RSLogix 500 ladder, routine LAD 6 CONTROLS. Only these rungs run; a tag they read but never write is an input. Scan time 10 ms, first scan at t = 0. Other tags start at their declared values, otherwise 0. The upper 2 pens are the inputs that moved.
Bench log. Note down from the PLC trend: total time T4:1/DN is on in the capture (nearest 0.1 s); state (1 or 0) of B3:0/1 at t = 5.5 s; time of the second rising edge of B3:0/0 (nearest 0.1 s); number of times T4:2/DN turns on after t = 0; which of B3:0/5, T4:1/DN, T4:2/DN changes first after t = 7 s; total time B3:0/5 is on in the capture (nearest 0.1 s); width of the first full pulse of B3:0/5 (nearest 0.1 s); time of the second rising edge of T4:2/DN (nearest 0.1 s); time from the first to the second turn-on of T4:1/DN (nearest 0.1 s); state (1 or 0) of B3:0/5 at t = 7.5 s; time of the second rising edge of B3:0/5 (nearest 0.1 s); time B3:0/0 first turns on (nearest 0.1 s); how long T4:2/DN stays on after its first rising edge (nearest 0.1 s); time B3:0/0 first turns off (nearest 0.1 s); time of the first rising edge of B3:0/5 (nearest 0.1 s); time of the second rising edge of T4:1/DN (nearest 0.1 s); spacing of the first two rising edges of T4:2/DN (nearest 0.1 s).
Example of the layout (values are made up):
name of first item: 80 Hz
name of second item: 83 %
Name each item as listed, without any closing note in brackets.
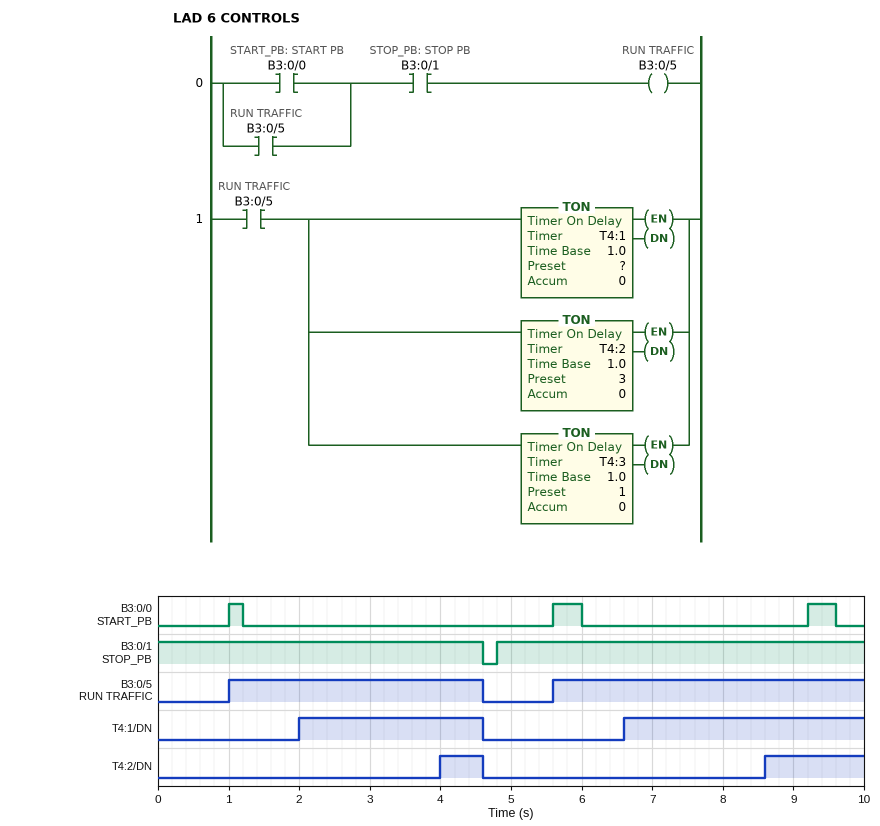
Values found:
total time T4:1/DN is on in the capture: 6.0 s
state (1 or 0) of B3:0/1 at t = 5.5 s: 1
time of the second rising edge of B3:0/0: 5.6 s
number of times T4:2/DN turns on after t = 0: 2
which of B3:0/5, T4:1/DN, T4:2/DN changes first after t = 7 s: T4:2/DN
total time B3:0/5 is on in the capture: 8.0 s
width of the first full pulse of B3:0/5: 3.6 s
time of the second rising edge of T4:2/DN: 8.6 s
time from the first to the second turn-on of T4:1/DN: 4.6 s
state (1 or 0) of B3:0/5 at t = 7.5 s: 1
time of the second rising edge of B3:0/5: 5.6 s
time B3:0/0 first turns on: 1.0 s
how long T4:2/DN stays on after its first rising edge: 0.6 s
time B3:0/0 first turns off: 1.2 s
time of the first rising edge of B3:0/5: 1.0 s
time of the second rising edge of T4:1/DN: 6.6 s
spacing of the first two rising edges of T4:2/DN: 4.6 s
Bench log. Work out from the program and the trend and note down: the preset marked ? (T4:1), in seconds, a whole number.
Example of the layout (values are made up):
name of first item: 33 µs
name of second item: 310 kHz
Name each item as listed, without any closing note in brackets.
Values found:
the preset marked ? (T4:1), in seconds, a whole number: 1 s
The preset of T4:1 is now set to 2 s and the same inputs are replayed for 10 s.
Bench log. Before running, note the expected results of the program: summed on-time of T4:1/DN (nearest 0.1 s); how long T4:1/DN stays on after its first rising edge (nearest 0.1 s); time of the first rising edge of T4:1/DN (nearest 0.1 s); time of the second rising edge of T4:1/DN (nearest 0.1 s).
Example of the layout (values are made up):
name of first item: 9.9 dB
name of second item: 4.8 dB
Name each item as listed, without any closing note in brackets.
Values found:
summed on-time of T4:1/DN: 4.0 s
how long T4:1/DN stays on after its first rising edge: 1.6 s
time of the first rising edge of T4:1/DN: 3.0 s
time of the second rising edge of T4:1/DN: 7.6 s
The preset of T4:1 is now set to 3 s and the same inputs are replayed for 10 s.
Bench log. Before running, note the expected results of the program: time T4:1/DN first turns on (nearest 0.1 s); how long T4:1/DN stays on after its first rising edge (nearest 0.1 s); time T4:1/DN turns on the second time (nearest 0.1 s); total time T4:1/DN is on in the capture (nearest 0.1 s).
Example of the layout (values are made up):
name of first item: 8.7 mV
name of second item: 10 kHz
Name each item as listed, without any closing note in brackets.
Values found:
time T4:1/DN first turns on: 4.0 s
how long T4:1/DN stays on after its first rising edge: 0.6 s
time T4:1/DN turns on the second time: 8.6 s
total time T4:1/DN is on in the capture: 2.0 s
